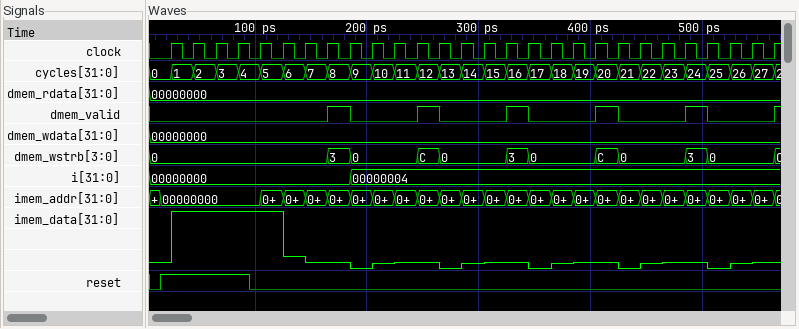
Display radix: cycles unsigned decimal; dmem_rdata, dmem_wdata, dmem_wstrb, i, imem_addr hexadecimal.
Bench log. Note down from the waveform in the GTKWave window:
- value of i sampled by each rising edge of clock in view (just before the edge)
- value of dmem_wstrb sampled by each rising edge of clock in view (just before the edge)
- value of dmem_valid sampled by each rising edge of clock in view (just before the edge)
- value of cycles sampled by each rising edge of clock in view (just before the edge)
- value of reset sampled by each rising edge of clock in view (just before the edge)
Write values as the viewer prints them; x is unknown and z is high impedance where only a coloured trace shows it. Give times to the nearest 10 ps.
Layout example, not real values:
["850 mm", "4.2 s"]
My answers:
["00000000, 00000000, 00000000, 00000000, 00000000, 00000000, 00000000, 00000000, 00000000, 00000004, 00000004, 00000004, 00000004, 00000004, 00000004, 00000004, 00000004, 00000004, 00000004, 00000004, 00000004, 00000004, 00000004, 00000004, 00000004, 00000004, 00000004, 00000004", "0, 0, 0, 0, 0, 0, 0, 0, 3, 0, 0, 0, C, 0, 0, 0, 3, 0, 0, 0, C, 0, 0, 0, 3, 0, 0, 0", "0 0 0 0 0 0 0 0 1 0 0 0 1 0 0 0 1 0 0 0 1 0 0 0 1 0 0 0", "0, 1, 2, 3, 4, 5, 6, 7, 8, 9, 10, 11, 12, 13, 14, 15, 16, 17, 18, 19, 20, 21, 22, 23, 24, 25, 26, 27", "1 1 1 1 0 0 0 0 0 0 0 0 0 0 0 0 0 0 0 0 0 0 0 0 0 0 0 0"]
